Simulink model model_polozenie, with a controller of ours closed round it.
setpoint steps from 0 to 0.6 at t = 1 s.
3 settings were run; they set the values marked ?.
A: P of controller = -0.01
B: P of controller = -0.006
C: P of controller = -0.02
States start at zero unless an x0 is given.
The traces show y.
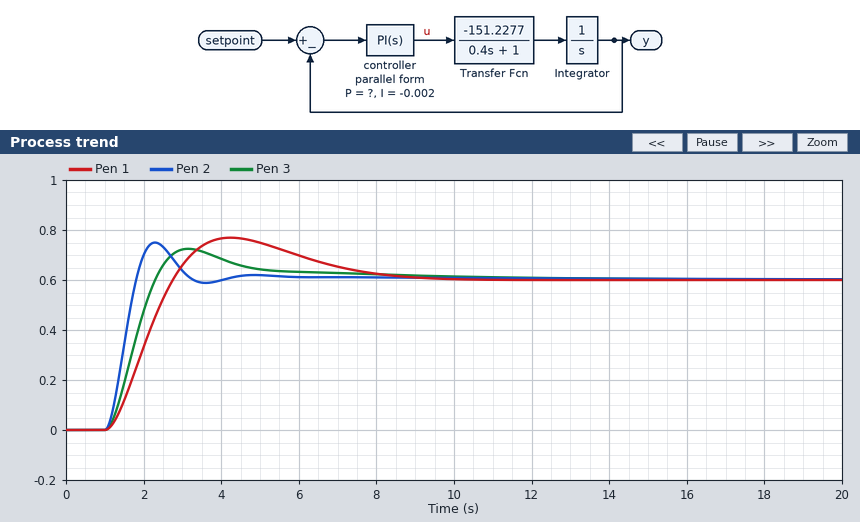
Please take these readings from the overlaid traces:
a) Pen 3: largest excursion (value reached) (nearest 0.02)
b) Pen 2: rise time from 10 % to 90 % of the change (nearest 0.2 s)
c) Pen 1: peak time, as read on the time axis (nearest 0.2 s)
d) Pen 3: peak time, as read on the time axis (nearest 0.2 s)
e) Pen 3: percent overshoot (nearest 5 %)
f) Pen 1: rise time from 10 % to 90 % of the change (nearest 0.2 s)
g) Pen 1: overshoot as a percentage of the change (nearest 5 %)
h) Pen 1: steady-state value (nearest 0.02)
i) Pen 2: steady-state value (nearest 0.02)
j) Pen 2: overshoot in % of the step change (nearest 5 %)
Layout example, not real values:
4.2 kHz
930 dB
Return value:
0.72
0.6 s
4.2 s
3.2 s
20 %
1.2 s
30 %
0.60
0.60
25 %
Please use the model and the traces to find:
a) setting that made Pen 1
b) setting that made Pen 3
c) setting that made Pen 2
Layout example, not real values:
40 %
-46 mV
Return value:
B
A
C
